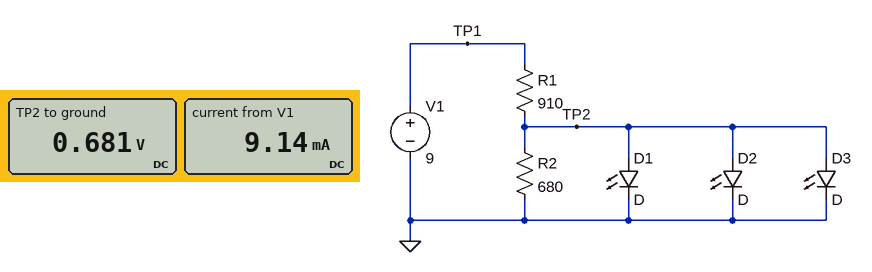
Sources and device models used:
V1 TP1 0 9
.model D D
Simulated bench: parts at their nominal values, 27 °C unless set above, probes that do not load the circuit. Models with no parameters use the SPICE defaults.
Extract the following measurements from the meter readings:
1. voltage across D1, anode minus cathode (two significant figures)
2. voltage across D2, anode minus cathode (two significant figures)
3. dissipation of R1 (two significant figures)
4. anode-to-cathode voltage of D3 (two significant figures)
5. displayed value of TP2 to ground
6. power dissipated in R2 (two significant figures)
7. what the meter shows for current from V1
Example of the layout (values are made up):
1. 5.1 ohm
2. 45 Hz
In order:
1. 680 mV
2. 680 mV
3. 76 mW
4. 680 mV
5. 0.681 V
6. 680 µW
7. 9.14 mA
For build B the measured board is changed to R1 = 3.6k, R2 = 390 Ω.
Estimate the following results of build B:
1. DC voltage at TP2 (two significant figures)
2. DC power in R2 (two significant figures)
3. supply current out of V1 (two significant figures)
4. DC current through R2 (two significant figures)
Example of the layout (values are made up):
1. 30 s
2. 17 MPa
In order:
1. 620 mV
2. 980 µW
3. 2.3 mA
4. 1.6 mA
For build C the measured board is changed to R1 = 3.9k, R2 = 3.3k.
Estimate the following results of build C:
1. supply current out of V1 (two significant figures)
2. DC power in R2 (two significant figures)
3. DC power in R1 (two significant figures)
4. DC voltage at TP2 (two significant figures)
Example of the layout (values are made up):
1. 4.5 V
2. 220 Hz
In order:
1. 2.1 mA
2. 130 µW
3. 18 mW
4. 640 mV
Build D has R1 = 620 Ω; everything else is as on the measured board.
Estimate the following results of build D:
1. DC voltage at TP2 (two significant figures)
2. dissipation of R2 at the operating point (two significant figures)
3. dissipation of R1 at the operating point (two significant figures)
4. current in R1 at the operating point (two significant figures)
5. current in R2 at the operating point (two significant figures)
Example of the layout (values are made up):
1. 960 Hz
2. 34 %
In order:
1. 690 mV
2. 700 µW
3. 110 mW
4. 13 mA
5. 1.0 mA
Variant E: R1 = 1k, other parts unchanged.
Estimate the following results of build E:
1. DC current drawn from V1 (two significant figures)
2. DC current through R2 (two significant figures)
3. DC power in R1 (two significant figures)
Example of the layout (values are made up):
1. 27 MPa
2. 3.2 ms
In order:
1. 8.3 mA
2. 1.0 mA
3. 69 mW
